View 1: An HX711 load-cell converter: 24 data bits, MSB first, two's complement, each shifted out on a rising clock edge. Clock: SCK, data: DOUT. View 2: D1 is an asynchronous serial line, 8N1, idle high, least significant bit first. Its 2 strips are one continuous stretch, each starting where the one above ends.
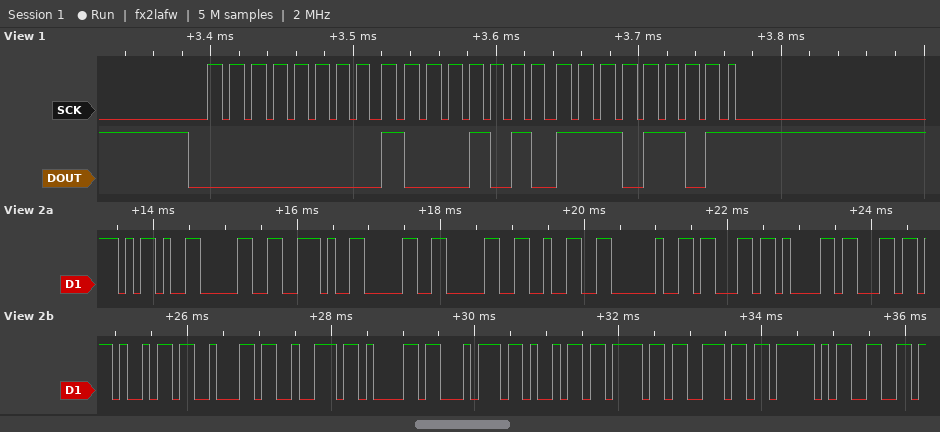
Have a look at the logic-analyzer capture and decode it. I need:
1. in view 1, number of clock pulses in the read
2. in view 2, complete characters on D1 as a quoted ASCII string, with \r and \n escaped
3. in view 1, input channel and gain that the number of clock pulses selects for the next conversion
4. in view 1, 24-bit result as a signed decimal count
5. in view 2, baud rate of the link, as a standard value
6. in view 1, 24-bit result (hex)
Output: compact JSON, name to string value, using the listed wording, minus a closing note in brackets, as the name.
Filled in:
{"in view 1, number of clock pulses in the read": "25", "in view 2, complete characters on D1 as a quoted ASCII string, with \\r and \\n escaped": "\"-0.002 calibration_f\"", "in view 1, input channel and gain that the number of clock pulses selects for the next conversion": "channel A, gain 128", "in view 1, 24-bit result as a signed decimal count": "35565", "in view 2, baud rate of the link, as a standard value": "9600 baud", "in view 1, 24-bit result": "0x008AED"}
